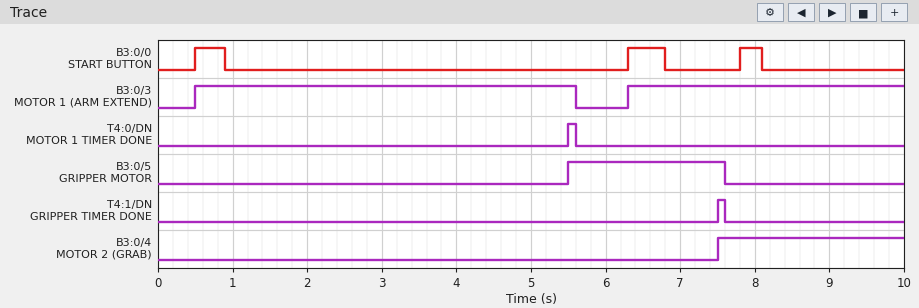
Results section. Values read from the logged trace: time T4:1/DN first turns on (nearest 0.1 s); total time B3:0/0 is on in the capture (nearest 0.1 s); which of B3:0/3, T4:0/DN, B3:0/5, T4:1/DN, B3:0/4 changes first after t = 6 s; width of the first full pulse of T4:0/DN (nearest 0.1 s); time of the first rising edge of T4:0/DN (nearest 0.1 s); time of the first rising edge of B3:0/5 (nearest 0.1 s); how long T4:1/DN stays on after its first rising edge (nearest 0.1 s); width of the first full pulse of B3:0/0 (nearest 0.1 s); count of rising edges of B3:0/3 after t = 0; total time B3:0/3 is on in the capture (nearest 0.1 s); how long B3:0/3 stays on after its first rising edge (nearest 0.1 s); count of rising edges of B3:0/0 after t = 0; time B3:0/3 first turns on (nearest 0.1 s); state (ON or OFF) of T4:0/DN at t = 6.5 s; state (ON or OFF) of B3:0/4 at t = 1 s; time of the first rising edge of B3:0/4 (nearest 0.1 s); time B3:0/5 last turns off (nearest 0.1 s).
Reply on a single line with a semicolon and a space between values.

7.5 s; 1.2 s; B3:0/3; 0.1 s; 5.5 s; 5.5 s; 0.1 s; 0.4 s; 2; 8.8 s; 5.1 s; 3; 0.5 s; OFF; OFF; 7.5 s; 7.6 s
